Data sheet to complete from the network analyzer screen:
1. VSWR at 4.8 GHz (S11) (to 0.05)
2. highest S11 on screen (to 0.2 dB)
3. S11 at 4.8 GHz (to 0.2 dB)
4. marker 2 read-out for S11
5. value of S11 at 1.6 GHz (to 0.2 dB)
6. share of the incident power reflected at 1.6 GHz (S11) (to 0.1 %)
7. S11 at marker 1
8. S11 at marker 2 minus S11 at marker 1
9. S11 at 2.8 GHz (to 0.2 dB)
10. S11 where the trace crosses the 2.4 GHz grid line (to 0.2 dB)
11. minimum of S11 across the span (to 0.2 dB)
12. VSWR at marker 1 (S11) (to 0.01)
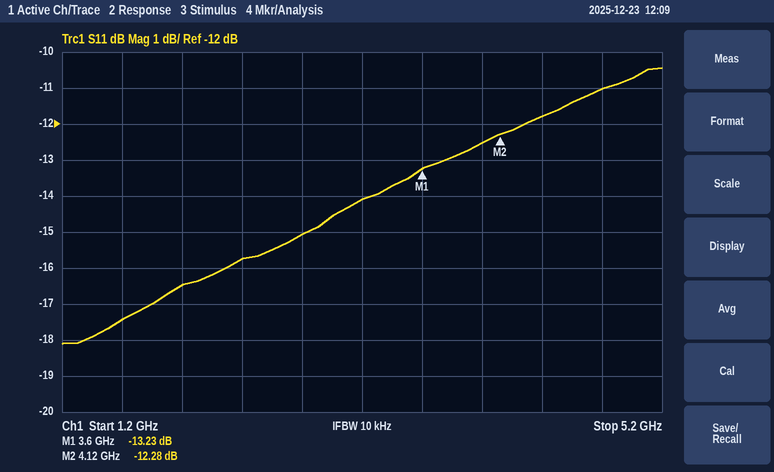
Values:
1.80
-10.4 dB
-11.0 dB
-12.28 dB
-17.4 dB
1.8 %
-13.23 dB
0.95 dB
-15.0 dB
-15.8 dB
-18.2 dB
1.56
